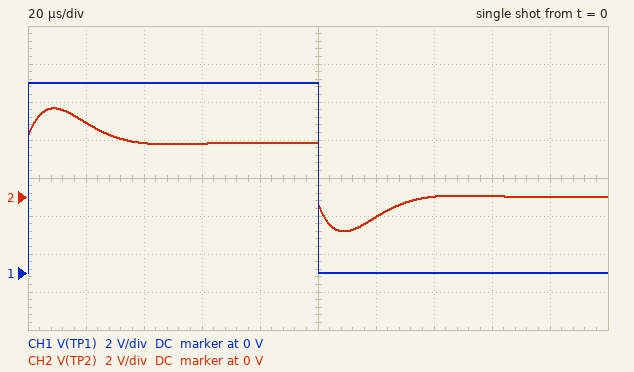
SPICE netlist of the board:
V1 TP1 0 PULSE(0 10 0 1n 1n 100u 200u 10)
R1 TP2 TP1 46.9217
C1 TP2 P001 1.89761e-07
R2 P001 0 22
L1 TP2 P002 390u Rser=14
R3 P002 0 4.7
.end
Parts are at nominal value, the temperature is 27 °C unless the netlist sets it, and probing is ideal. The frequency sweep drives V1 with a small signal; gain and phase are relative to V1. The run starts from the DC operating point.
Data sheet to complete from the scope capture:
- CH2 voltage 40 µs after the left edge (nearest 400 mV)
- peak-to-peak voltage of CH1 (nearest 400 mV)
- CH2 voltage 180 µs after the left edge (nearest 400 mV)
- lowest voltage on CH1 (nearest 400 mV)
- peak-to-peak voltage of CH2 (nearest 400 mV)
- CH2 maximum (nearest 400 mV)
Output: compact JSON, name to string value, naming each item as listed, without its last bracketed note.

{"CH2 voltage 40 µs after the left edge": "2.8 V", "peak-to-peak voltage of CH1": "10.0 V", "CH2 voltage 180 µs after the left edge": "0 V", "lowest voltage on CH1": "0 V", "peak-to-peak voltage of CH2": "6.4 V", "CH2 maximum": "4.8 V"}
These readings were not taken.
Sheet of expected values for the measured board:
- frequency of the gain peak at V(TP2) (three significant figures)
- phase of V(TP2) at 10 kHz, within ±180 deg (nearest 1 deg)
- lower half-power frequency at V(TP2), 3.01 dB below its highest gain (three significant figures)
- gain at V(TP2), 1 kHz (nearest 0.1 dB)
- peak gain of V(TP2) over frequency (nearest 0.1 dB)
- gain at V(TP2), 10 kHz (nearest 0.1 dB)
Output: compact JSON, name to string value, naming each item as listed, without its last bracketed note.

{"frequency of the gain peak at V(TP2)": "18.5 kHz", "phase of V(TP2) at 10 kHz, within ±180 deg": "18 deg", "lower half-power frequency at V(TP2), 3.01 dB below its highest gain": "7.49 kHz", "gain at V(TP2), 1 kHz": "-10.8 dB", "peak gain of V(TP2) over frequency": "-5.0 dB", "gain at V(TP2), 10 kHz": "-6.7 dB"}
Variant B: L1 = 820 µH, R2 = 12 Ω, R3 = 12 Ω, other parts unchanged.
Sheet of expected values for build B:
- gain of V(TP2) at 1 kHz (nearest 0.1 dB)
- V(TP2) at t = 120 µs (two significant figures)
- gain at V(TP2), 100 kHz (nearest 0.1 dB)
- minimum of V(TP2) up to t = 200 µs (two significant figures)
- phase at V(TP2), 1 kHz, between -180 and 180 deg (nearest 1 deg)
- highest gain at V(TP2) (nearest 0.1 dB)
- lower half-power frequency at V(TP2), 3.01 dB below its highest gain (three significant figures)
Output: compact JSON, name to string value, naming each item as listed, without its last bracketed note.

{"gain of V(TP2) at 1 kHz": "-8.8 dB", "V(TP2) at t = 120 µs": "-2.3 V", "gain at V(TP2), 100 kHz": "-12.1 dB", "minimum of V(TP2) up to t = 200 µs": "-2.5 V", "phase at V(TP2), 1 kHz, between -180 and 180 deg": "6 deg", "highest gain at V(TP2)": "-2.7 dB", "lower half-power frequency at V(TP2), 3.01 dB below its highest gain": "5.54 kHz"}
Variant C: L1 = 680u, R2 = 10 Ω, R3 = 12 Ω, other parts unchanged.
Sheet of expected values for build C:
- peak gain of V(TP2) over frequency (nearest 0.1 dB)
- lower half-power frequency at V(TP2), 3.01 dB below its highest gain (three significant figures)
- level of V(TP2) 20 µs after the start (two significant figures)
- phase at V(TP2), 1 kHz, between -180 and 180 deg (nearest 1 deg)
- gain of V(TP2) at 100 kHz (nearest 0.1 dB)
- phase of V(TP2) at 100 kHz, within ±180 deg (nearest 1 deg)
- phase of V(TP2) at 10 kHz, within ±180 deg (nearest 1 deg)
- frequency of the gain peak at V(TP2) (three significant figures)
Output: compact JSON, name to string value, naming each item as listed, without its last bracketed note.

{"peak gain of V(TP2) over frequency": "-3.0 dB", "lower half-power frequency at V(TP2), 3.01 dB below its highest gain": "6.15 kHz", "level of V(TP2) 20 µs after the start": "5.6 V", "phase at V(TP2), 1 kHz, between -180 and 180 deg": "5 deg", "gain of V(TP2) at 100 kHz": "-12.8 dB", "phase of V(TP2) at 100 kHz, within ±180 deg": "-30 deg", "phase of V(TP2) at 10 kHz, within ±180 deg": "9 deg", "frequency of the gain peak at V(TP2)": "15.0 kHz"}
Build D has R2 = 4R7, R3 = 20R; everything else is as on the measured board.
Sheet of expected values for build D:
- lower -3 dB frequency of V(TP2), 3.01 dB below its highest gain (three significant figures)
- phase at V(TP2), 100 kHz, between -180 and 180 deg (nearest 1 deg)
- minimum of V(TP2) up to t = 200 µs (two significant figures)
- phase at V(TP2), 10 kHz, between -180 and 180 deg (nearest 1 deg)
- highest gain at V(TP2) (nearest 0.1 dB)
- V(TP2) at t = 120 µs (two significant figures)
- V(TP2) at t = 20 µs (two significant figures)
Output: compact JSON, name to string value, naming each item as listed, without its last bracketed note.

{"lower -3 dB frequency of V(TP2), 3.01 dB below its highest gain": "3.22 kHz", "phase at V(TP2), 100 kHz, between -180 and 180 deg": "-50 deg", "minimum of V(TP2) up to t = 200 µs": "-1.3 V", "phase at V(TP2), 10 kHz, between -180 and 180 deg": "3 deg", "highest gain at V(TP2)": "-4.3 dB", "V(TP2) at t = 120 µs": "-870 mV", "V(TP2) at t = 20 µs": "5.1 V"}
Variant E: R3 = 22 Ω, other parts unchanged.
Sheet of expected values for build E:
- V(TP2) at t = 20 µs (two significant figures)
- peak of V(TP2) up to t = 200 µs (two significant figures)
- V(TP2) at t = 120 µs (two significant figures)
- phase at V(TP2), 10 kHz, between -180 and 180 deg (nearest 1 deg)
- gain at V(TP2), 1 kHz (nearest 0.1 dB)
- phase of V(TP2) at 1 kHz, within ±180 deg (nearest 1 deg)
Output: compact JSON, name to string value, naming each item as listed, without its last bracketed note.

{"V(TP2) at t = 20 µs": "4.8 V", "peak of V(TP2) up to t = 200 µs": "5.0 V", "V(TP2) at t = 120 µs": "-460 mV", "phase at V(TP2), 10 kHz, between -180 and 180 deg": "2 deg", "gain at V(TP2), 1 kHz": "-7.2 dB", "phase of V(TP2) at 1 kHz, within ±180 deg": "1 deg"}
